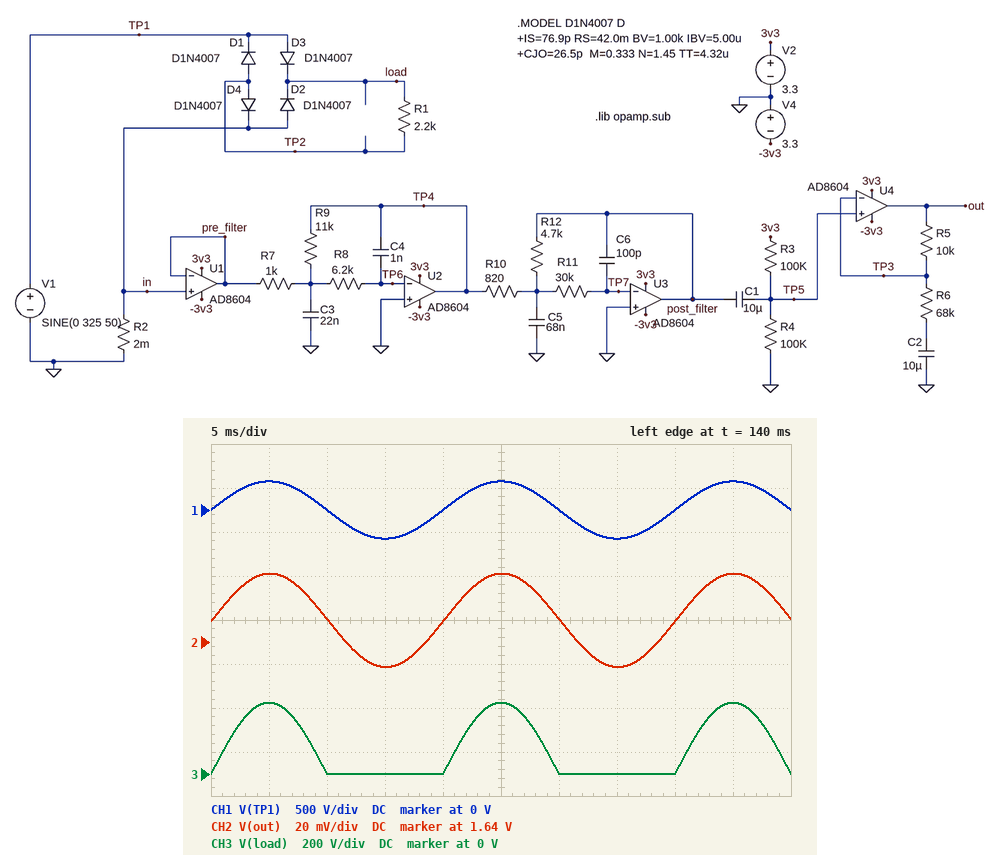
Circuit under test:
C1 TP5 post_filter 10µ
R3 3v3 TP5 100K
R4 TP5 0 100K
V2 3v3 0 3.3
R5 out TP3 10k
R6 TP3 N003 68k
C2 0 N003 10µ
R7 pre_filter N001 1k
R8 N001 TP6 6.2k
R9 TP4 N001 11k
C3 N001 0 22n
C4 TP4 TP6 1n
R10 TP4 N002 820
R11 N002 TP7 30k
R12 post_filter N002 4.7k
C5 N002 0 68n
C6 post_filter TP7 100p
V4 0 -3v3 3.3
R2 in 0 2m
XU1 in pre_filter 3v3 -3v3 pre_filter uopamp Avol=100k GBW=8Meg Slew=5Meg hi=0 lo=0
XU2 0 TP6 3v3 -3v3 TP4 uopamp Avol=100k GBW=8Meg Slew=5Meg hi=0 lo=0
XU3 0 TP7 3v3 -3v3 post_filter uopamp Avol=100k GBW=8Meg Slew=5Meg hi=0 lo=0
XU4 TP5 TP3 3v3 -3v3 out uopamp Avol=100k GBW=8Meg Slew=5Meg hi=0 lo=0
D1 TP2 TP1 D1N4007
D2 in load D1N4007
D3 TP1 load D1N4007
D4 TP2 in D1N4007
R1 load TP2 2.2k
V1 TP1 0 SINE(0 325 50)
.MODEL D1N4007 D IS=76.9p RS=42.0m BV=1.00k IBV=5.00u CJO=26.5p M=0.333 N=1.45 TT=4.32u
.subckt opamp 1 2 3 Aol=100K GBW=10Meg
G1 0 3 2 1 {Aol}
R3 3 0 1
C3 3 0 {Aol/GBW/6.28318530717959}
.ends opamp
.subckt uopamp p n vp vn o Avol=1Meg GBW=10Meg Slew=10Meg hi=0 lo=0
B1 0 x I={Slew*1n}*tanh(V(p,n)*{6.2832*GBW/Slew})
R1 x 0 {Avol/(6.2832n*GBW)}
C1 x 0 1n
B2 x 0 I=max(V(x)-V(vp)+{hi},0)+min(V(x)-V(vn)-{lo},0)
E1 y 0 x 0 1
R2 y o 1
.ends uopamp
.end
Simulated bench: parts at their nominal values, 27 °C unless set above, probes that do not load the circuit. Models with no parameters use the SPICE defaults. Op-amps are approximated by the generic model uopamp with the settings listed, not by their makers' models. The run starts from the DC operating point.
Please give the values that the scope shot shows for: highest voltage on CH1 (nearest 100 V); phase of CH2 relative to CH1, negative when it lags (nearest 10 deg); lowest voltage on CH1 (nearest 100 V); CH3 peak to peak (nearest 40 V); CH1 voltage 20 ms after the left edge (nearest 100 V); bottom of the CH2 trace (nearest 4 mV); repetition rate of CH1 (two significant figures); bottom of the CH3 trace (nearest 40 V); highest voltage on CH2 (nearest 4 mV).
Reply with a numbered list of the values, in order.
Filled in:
1. 300 V
2. 0 deg
3. -300 V
4. 320 V
5. 0 V
6. 1.628 V
7. 50 Hz
8. 0 V
9. 1.672 V
